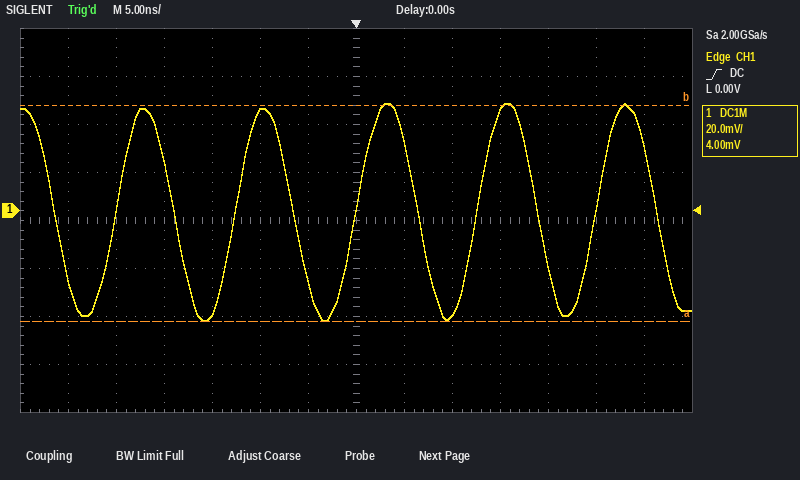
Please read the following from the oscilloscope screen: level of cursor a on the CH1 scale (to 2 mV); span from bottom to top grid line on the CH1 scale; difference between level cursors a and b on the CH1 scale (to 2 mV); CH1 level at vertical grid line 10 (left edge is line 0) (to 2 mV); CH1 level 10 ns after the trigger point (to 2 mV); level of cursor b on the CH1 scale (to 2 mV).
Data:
-46 mV
160 mV
90 mV
42 mV
-44 mV
44 mV
